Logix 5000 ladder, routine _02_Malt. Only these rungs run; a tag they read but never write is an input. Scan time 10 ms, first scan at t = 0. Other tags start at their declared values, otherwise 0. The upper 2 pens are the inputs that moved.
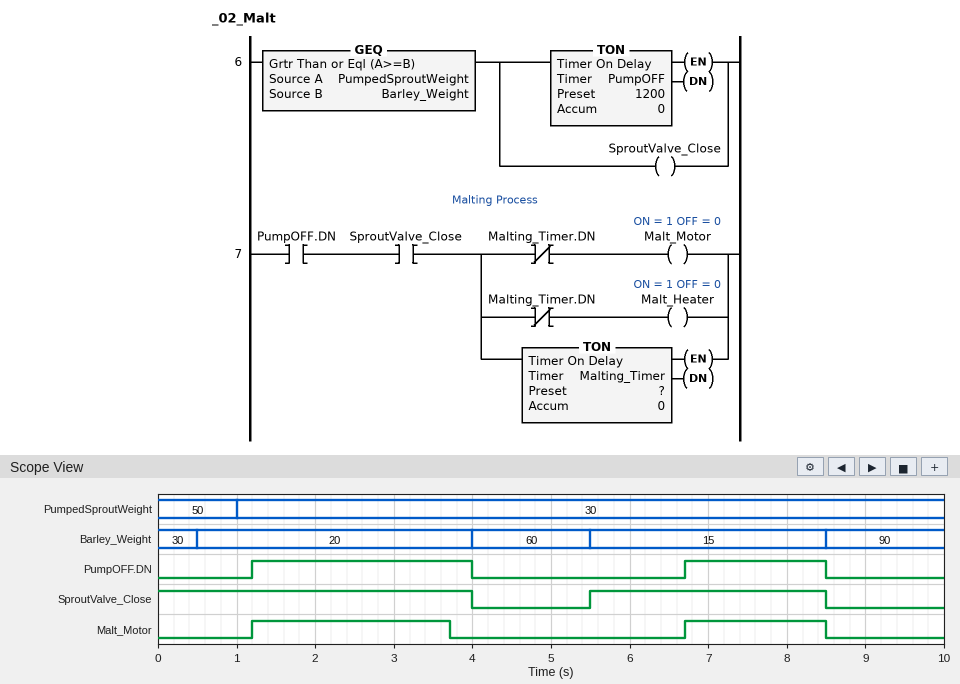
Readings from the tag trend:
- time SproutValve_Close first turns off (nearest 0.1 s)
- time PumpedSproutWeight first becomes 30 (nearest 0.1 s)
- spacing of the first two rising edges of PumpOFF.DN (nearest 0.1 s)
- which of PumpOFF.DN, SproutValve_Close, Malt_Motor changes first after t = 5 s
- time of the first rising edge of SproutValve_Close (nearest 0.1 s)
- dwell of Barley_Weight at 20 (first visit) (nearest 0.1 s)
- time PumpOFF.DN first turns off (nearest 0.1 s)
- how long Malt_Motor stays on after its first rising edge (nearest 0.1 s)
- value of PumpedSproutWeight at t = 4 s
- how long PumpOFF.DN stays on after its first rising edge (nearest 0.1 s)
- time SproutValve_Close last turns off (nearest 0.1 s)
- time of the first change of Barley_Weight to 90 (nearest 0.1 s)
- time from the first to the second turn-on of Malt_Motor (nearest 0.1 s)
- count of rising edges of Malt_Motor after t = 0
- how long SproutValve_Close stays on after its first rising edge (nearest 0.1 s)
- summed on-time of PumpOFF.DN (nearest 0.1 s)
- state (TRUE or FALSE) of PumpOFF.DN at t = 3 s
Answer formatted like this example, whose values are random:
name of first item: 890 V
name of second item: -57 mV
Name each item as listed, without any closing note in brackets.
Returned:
time SproutValve_Close first turns off: 4.0 s
time PumpedSproutWeight first becomes 30: 1.0 s
spacing of the first two rising edges of PumpOFF.DN: 5.5 s
which of PumpOFF.DN, SproutValve_Close, Malt_Motor changes first after t = 5 s: SproutValve_Close
time of the first rising edge of SproutValve_Close: 5.5 s
dwell of Barley_Weight at 20 (first visit): 3.5 s
time PumpOFF.DN first turns off: 4.0 s
how long Malt_Motor stays on after its first rising edge: 2.5 s
value of PumpedSproutWeight at t = 4 s: 30
how long PumpOFF.DN stays on after its first rising edge: 2.8 s
time SproutValve_Close last turns off: 8.5 s
time of the first change of Barley_Weight to 90: 8.5 s
time from the first to the second turn-on of Malt_Motor: 5.5 s
count of rising edges of Malt_Motor after t = 0: 2
how long SproutValve_Close stays on after its first rising edge: 3.0 s
summed on-time of PumpOFF.DN: 4.6 s
state (TRUE or FALSE) of PumpOFF.DN at t = 3 s: TRUE
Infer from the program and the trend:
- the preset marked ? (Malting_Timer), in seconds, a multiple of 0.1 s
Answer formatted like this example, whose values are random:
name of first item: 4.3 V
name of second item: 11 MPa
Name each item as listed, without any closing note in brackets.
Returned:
the preset marked ? (Malting_Timer), in seconds, a multiple of 0.1 s: 2.5 s
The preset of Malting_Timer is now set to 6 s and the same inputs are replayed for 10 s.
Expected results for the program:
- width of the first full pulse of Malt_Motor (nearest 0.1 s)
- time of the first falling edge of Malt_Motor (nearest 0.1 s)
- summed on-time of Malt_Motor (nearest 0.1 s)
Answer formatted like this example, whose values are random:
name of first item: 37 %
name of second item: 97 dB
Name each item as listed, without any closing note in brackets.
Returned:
width of the first full pulse of Malt_Motor: 2.8 s
time of the first falling edge of Malt_Motor: 4.0 s
summed on-time of Malt_Motor: 4.6 s
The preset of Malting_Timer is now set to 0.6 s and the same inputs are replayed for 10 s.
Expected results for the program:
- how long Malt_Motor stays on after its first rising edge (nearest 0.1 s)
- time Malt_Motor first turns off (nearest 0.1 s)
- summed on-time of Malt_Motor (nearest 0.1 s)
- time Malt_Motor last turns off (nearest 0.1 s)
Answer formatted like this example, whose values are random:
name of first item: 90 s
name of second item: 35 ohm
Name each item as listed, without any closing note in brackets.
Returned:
how long Malt_Motor stays on after its first rising edge: 0.6 s
time Malt_Motor first turns off: 1.8 s
summed on-time of Malt_Motor: 1.2 s
time Malt_Motor last turns off: 7.3 s
